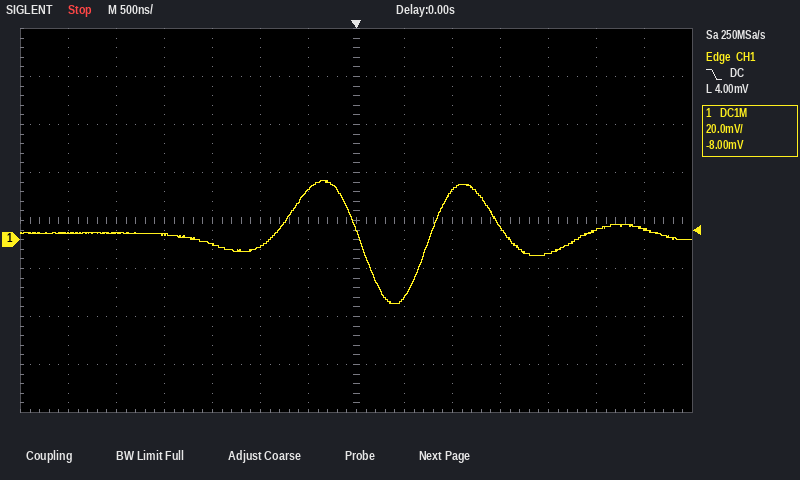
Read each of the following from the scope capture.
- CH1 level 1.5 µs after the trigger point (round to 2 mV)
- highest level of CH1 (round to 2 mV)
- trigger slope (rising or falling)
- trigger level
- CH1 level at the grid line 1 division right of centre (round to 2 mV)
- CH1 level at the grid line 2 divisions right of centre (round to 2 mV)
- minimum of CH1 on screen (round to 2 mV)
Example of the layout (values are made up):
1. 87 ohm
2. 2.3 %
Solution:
1. 6 mV
2. 24 mV
3. falling
4. 4.00 mV
5. -24 mV
6. 20 mV
7. -26 mV
